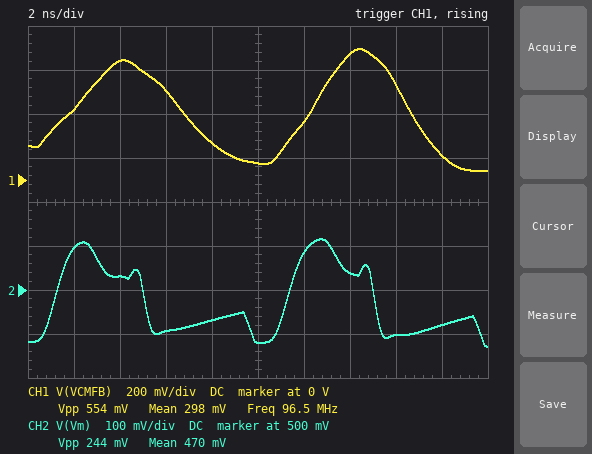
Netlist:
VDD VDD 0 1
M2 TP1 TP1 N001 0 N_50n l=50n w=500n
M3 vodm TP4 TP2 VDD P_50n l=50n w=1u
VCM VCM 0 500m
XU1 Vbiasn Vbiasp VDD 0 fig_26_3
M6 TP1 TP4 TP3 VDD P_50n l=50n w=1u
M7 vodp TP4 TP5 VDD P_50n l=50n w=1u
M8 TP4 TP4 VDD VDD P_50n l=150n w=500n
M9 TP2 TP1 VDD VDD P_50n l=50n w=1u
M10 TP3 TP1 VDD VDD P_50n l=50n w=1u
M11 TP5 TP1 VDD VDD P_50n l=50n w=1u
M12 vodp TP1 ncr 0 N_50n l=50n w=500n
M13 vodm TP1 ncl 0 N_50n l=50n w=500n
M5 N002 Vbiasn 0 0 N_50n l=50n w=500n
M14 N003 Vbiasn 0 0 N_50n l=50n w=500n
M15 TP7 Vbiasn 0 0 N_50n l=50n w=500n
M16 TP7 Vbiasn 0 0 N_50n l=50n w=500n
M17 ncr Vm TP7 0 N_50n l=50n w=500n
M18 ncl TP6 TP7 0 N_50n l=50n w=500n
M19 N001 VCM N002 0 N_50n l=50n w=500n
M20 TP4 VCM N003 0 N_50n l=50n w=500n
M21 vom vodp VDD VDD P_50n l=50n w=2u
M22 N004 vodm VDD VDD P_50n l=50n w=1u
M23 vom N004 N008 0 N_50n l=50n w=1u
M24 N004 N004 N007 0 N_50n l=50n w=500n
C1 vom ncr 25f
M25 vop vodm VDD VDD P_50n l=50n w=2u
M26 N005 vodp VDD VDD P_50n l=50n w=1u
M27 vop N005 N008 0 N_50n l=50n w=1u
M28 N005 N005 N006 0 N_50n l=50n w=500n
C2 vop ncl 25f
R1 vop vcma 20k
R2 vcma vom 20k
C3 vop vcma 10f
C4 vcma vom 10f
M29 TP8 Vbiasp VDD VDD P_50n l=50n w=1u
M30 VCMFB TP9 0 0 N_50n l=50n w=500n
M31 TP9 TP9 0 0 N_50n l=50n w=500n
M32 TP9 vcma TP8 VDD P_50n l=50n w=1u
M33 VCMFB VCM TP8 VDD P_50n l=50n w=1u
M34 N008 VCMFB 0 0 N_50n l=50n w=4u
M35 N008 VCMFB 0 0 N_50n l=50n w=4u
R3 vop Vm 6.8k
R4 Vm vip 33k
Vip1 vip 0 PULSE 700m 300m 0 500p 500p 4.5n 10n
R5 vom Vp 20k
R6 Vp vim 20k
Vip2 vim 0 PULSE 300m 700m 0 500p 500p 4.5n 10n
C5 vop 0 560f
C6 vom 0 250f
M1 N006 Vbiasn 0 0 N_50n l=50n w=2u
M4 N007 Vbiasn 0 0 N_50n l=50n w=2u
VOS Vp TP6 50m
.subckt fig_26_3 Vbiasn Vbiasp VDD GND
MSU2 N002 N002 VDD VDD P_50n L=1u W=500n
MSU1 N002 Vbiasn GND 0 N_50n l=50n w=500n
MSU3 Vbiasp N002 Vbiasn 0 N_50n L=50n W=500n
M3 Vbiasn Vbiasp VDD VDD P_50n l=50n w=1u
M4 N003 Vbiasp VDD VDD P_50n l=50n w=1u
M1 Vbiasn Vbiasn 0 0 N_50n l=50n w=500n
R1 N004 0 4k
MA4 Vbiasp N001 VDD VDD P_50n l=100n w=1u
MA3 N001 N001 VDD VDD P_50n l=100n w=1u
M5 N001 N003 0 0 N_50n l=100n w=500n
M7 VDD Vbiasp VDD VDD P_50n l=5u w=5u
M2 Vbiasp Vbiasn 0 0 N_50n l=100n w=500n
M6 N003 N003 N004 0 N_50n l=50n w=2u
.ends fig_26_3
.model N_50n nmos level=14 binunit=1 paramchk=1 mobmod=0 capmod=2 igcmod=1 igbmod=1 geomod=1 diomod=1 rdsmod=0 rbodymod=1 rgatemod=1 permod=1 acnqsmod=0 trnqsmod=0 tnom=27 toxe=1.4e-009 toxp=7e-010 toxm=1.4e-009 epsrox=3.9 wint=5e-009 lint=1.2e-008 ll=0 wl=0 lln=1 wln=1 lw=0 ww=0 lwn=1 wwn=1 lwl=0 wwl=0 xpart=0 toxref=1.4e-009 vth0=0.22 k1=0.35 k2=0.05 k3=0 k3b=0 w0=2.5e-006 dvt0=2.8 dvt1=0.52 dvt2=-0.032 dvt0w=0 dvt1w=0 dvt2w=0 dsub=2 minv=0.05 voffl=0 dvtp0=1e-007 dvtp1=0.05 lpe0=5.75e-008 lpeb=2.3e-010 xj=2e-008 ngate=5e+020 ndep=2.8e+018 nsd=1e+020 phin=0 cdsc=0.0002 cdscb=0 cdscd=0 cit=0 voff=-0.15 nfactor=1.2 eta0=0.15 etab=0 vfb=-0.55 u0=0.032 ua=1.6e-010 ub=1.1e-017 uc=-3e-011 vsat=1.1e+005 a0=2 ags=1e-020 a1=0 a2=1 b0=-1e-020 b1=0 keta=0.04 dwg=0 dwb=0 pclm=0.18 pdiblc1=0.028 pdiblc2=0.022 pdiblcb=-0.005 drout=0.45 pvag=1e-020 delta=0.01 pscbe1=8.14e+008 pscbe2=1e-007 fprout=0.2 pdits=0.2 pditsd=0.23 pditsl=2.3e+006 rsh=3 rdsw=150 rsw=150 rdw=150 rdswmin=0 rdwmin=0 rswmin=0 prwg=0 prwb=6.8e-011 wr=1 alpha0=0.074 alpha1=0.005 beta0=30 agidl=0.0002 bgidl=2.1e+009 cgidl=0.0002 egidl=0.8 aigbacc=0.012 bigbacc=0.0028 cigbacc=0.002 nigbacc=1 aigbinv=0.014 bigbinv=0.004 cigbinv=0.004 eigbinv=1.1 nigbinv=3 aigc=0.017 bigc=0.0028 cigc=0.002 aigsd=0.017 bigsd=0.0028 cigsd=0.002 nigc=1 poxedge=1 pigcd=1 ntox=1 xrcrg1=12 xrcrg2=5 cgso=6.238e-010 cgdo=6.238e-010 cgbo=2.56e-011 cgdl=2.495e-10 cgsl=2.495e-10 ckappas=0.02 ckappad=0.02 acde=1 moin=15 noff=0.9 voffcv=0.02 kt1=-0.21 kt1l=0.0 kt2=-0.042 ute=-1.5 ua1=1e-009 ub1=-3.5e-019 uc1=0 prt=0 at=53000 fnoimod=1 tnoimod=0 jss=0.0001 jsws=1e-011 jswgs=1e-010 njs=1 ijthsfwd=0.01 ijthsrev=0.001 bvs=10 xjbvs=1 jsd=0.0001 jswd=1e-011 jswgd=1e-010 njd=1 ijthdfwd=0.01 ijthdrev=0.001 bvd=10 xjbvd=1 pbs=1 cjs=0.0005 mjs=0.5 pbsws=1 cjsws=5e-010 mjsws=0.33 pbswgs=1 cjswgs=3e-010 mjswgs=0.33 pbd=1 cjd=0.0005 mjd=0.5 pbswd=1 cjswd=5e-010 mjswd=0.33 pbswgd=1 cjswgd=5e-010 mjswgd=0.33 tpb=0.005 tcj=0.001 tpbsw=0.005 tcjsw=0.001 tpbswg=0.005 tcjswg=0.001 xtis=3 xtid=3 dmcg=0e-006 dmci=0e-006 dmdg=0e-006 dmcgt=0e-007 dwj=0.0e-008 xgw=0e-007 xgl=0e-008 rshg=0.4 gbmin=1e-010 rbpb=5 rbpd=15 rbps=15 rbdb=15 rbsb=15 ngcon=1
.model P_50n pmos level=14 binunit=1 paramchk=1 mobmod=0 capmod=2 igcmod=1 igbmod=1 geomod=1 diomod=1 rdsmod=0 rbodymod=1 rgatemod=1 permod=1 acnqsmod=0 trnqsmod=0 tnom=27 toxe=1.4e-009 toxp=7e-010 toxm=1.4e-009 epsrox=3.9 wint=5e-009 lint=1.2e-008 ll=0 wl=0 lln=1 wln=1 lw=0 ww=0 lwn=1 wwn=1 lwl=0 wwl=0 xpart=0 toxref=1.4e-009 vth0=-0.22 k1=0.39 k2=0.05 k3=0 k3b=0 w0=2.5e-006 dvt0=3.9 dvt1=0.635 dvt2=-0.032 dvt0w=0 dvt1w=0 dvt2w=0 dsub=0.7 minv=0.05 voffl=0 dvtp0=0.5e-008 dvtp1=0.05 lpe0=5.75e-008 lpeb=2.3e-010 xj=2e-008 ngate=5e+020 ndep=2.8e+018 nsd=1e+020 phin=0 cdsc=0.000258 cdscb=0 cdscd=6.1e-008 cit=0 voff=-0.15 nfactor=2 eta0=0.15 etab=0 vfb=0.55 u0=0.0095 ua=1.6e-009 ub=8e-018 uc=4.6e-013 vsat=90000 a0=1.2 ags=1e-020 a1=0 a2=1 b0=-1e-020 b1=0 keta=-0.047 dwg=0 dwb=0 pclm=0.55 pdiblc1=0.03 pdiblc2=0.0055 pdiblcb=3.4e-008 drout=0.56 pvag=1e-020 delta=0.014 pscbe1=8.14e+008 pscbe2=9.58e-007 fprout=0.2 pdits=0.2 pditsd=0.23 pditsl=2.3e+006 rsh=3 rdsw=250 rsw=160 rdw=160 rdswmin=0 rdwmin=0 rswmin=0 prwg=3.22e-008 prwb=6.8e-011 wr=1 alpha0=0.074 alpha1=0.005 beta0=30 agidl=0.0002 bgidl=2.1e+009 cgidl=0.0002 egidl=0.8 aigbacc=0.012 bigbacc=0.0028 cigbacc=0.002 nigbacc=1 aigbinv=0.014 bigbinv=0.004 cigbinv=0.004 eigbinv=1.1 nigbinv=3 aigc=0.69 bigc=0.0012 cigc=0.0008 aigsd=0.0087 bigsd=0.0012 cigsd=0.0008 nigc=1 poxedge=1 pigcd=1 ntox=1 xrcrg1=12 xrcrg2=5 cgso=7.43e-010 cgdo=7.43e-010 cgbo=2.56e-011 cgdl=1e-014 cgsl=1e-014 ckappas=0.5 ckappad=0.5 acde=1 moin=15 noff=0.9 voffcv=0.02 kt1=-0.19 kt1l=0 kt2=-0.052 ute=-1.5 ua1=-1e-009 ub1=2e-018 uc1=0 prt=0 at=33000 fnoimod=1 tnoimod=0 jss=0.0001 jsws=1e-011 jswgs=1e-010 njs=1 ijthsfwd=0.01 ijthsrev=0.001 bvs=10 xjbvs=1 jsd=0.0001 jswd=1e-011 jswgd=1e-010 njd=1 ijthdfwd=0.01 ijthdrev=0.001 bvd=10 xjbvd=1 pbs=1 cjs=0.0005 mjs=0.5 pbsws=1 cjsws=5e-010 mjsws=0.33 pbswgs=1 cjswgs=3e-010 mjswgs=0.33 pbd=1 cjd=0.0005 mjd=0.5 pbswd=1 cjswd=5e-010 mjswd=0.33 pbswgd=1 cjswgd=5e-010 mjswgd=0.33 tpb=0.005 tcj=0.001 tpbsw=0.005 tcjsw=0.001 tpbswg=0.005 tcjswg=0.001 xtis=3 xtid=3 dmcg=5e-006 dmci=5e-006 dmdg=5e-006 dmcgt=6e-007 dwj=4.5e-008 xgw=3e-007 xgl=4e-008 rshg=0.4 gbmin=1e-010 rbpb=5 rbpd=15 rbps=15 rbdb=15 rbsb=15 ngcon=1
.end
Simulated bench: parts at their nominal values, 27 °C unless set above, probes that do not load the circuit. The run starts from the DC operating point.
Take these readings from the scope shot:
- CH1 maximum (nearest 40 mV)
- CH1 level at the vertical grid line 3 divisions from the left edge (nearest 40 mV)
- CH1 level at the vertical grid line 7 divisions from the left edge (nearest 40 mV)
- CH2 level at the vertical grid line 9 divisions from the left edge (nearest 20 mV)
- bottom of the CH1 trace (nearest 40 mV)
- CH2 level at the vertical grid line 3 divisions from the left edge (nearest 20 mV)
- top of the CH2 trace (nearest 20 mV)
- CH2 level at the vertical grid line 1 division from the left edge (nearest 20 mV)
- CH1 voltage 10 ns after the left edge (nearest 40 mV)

600 mV
400 mV
560 mV
420 mV
40 mV
400 mV
620 mV
600 mV
80 mV
